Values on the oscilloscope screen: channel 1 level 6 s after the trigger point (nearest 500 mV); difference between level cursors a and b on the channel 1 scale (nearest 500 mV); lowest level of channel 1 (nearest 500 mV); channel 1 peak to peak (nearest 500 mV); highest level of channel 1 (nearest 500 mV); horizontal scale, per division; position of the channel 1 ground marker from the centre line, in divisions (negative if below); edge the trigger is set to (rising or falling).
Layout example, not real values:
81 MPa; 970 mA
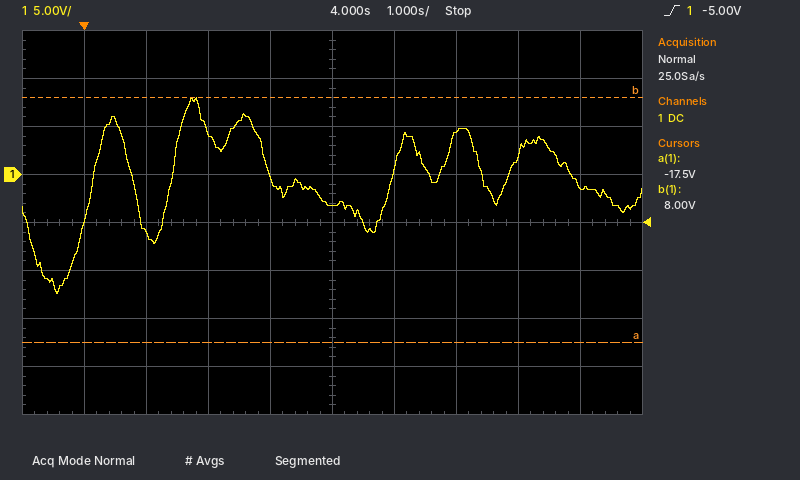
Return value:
4.5 V; 25.5 V; -12.5 V; 20.5 V; 8.0 V; 1 s; +1.0 div; rising
